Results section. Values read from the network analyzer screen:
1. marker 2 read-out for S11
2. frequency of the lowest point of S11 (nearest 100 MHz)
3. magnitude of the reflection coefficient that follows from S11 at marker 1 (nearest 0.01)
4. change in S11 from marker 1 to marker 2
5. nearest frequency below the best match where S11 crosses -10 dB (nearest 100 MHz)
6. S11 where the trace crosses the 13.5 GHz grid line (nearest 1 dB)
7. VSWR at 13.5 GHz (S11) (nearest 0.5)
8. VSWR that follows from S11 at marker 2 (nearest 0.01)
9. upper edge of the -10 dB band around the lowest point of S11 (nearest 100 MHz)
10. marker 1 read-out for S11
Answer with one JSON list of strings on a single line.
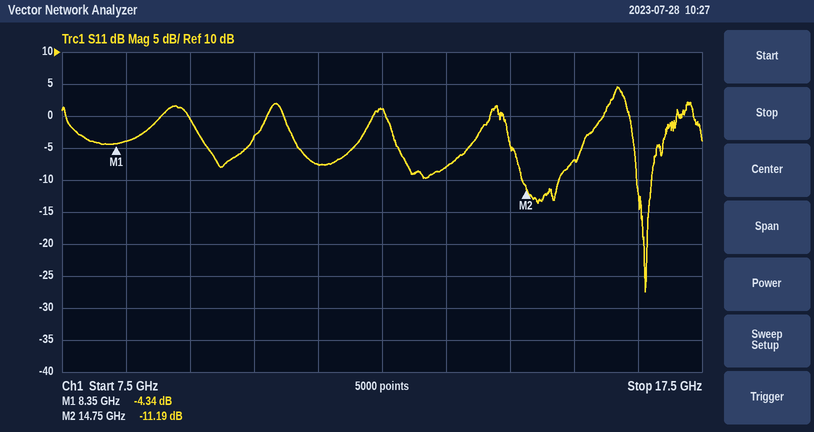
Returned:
["-11.19 dB", "16.6 GHz", "0.61", "-6.85 dB", "16.5 GHz", "-8 dB", "2.5", "1.76", "16.7 GHz", "-4.34 dB"]
